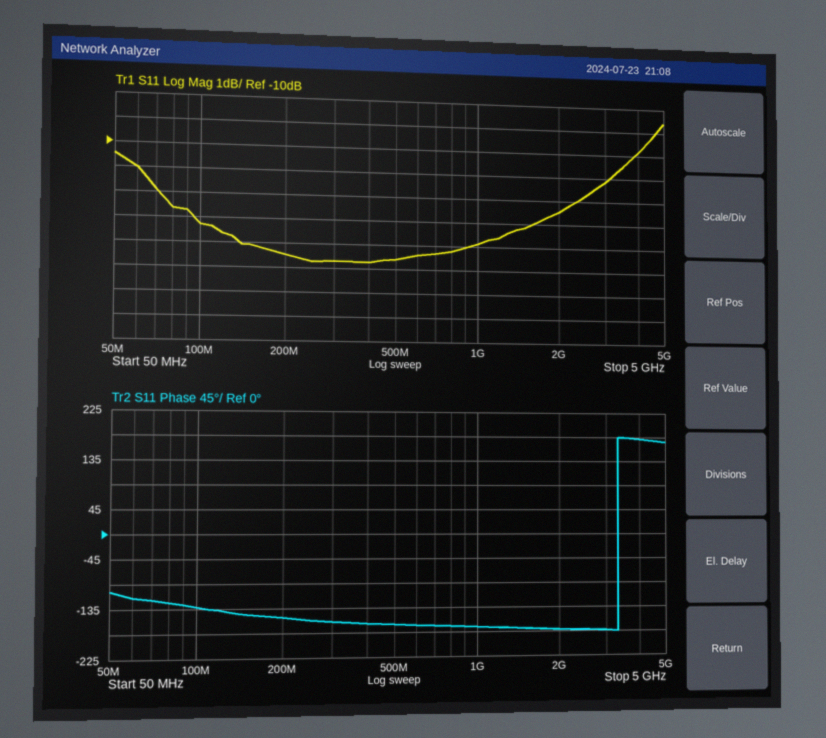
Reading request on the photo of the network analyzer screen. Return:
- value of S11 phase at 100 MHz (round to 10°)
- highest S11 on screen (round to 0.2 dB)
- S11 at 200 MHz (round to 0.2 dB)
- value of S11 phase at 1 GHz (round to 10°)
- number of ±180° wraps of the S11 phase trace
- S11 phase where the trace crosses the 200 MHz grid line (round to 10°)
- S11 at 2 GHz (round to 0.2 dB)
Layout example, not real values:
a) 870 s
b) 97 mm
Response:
a) -130°
b) -8.6 dB
c) -14.4 dB
d) -170°
e) 1
f) -150°
g) -12.4 dB
